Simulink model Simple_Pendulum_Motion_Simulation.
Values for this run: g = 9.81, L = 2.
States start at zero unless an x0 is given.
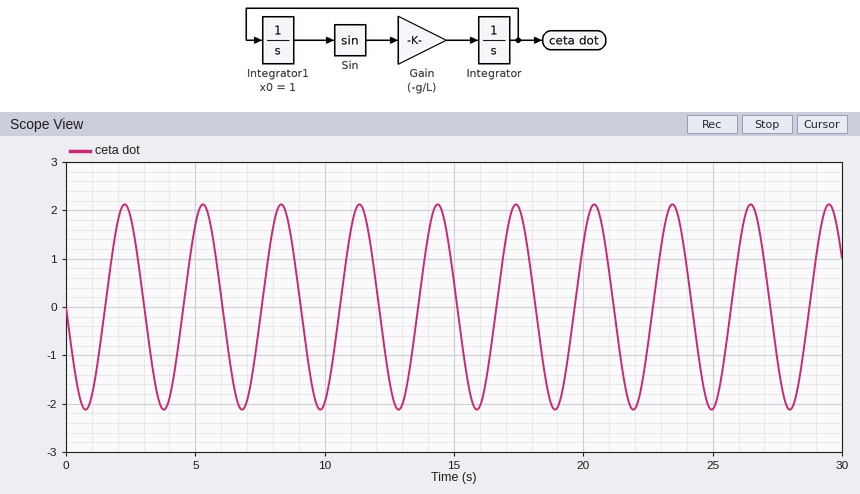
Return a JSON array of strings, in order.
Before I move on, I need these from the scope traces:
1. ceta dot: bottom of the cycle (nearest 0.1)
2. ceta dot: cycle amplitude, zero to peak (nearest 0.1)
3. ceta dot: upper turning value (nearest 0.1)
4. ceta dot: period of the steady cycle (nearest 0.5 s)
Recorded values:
["-2.1", "2.1", "2.1", "3.0 s"]
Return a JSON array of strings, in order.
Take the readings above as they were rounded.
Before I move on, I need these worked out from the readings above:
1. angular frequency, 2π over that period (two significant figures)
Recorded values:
["2.1 rad/s"]
